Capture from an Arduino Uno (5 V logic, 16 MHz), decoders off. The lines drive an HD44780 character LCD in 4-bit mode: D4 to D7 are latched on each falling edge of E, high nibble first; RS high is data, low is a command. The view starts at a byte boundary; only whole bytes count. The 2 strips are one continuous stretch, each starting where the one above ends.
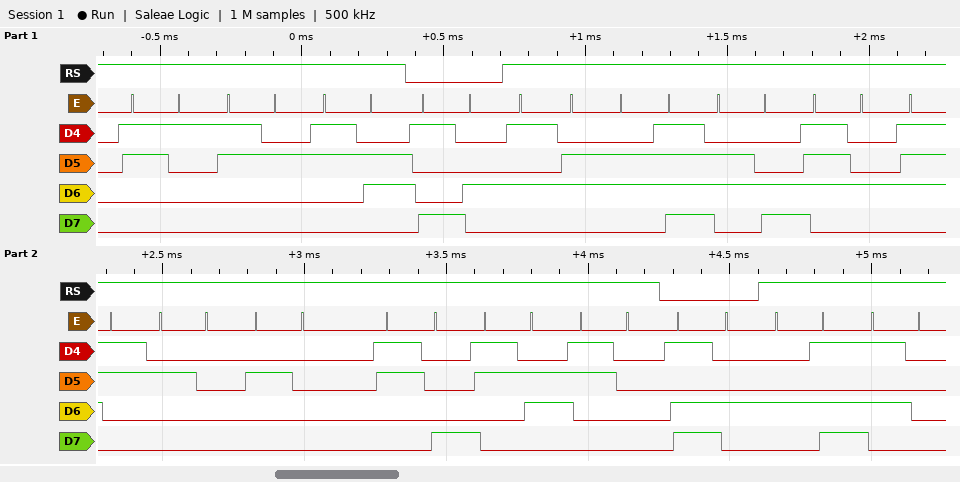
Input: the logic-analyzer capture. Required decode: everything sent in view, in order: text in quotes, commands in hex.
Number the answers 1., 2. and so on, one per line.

1. "126" 0x94 "Volts  860" 0xD4 "MP"
